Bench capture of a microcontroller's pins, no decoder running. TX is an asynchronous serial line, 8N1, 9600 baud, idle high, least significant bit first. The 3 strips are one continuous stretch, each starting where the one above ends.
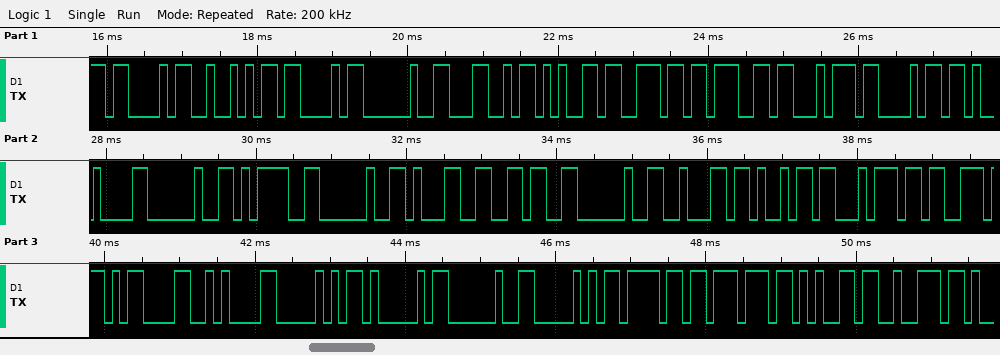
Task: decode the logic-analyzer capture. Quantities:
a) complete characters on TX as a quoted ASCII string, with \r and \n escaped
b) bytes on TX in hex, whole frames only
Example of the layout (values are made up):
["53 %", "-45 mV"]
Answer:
["\"CRC Length\\t = 16 bits\\r\\nPA Power\"", "43 52 43 20 4C 65 6E 67 74 68 09 20 3D 20 31 36 20 62 69 74 73 0D 0A 50 41 20 50 6F 77 65 72"]
